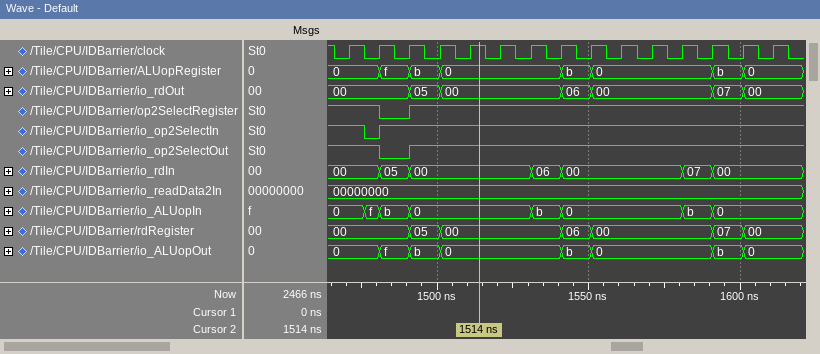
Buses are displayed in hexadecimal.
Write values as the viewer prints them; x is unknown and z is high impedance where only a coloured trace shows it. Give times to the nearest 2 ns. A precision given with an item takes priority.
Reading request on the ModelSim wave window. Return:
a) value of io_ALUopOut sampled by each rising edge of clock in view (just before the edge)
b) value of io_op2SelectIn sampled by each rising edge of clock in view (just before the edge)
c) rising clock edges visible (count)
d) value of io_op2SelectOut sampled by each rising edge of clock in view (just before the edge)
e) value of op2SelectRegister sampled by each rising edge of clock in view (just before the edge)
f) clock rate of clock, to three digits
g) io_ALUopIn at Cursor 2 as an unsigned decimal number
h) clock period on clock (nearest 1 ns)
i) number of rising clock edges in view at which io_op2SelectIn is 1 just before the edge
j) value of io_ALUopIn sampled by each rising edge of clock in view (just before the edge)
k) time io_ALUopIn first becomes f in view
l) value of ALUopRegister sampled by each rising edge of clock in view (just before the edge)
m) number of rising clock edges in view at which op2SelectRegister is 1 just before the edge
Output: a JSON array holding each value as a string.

["0, 0, f, b, 0, 0, 0, 0, b, 0, 0, 0, 0, b, 0", "1 0 1 1 1 1 1 1 1 1 1 1 1 1 1", "15", "1 1 0 1 1 1 1 1 1 1 1 1 1 1 1", "1 1 0 1 1 1 1 1 1 1 1 1 1 1 1", "100 MHz", "0", "10 ns", "14", "0, f, b, 0, 0, 0, 0, b, 0, 0, 0, 0, b, 0, 0", "1476 ns", "0, 0, f, b, 0, 0, 0, 0, b, 0, 0, 0, 0, b, 0", "14"]
